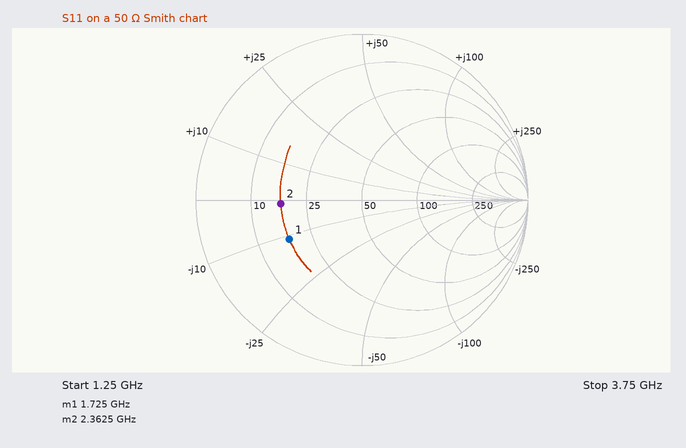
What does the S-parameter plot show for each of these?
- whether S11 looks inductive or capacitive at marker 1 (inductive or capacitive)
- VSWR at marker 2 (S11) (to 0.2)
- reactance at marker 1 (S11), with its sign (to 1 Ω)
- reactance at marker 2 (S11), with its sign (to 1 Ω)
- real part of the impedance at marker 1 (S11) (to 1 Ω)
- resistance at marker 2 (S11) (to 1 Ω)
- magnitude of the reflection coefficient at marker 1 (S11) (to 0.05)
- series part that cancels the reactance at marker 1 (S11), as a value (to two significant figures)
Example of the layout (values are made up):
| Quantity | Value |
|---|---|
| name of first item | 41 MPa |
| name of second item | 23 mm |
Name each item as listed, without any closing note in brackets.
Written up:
| Quantity | Value |
|---|---|
| whether S11 looks inductive or capacitive at marker 1 | capacitive |
| VSWR at marker 2 (S11) | 3.0 |
| reactance at marker 1 (S11), with its sign | -11 Ω |
| reactance at marker 2 (S11), with its sign | -1 Ω |
| real part of the impedance at marker 1 (S11) | 18 Ω |
| resistance at marker 2 (S11) | 17 Ω |
| magnitude of the reflection coefficient at marker 1 (S11) | 0.50 |
| series part that cancels the reactance at marker 1 (S11), as a value | 1.0 nH |
